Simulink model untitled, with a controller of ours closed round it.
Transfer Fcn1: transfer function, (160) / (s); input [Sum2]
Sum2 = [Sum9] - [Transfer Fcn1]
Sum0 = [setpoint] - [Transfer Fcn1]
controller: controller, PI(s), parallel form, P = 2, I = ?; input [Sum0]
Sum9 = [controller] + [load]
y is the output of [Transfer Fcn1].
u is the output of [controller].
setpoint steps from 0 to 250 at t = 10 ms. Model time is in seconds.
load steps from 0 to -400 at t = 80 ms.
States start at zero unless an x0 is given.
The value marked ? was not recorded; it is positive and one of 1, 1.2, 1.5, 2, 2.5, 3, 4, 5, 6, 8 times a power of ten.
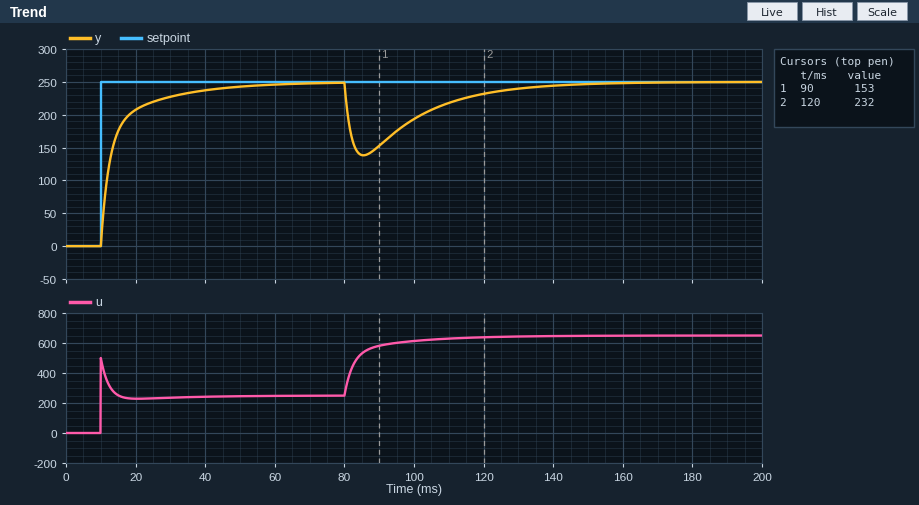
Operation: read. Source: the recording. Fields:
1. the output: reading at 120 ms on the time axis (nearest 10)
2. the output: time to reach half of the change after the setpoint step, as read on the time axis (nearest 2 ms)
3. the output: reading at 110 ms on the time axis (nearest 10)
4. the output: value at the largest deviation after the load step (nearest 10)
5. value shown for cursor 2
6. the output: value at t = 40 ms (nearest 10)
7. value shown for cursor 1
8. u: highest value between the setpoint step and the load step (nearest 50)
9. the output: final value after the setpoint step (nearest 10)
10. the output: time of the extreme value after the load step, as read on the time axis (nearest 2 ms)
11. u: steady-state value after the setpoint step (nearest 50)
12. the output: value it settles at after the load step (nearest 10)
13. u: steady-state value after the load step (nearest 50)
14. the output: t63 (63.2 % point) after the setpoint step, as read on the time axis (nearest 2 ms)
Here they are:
230
12 ms
220
140
232
240
153
500
250
86 ms
250
250
650
14 ms
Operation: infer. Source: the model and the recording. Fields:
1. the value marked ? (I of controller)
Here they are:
150
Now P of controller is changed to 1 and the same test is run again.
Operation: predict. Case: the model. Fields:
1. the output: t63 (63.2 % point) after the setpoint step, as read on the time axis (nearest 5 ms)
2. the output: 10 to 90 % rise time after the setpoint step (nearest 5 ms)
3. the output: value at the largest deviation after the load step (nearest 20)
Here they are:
15 ms
15 ms
100
